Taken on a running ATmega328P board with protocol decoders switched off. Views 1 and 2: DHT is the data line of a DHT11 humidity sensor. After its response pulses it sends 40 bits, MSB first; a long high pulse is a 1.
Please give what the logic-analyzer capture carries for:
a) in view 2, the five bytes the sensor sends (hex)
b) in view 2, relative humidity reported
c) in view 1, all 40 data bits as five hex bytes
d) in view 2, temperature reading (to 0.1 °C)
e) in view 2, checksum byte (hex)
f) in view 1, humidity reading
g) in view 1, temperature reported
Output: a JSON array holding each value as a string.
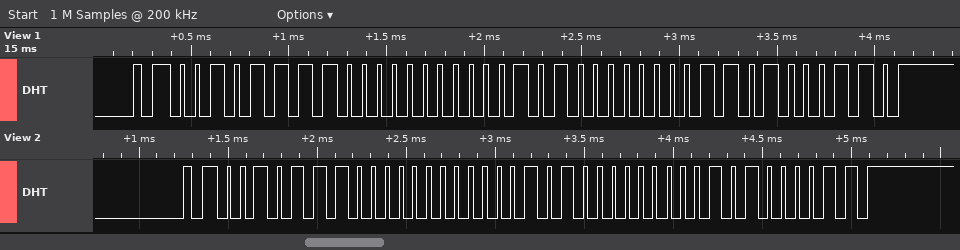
["2E 00 14 01 43", "46 %", "2F 00 14 03 46", "20.1 °C", "0x43", "47 %", "20.3 °C"]
